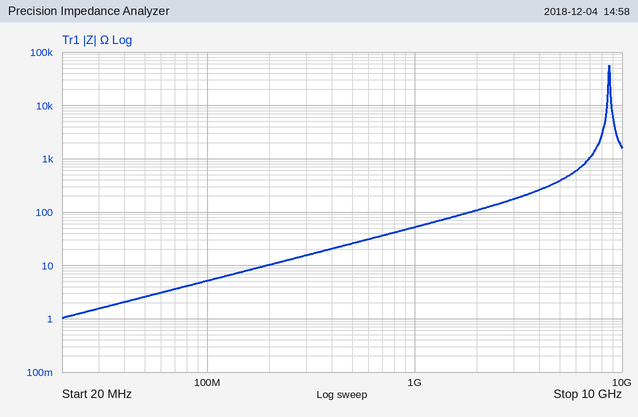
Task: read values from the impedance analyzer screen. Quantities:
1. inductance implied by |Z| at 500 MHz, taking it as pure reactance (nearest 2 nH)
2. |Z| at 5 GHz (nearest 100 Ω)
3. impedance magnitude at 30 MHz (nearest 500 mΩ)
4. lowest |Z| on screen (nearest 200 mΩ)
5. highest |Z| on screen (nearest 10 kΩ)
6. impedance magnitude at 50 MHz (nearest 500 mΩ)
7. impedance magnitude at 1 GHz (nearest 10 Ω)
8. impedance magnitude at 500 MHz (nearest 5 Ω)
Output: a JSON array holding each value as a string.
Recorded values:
["8 nH", "400 Ω", "1.5 Ω", "1.0 Ω", "60 kΩ", "2.5 Ω", "50 Ω", "25 Ω"]
